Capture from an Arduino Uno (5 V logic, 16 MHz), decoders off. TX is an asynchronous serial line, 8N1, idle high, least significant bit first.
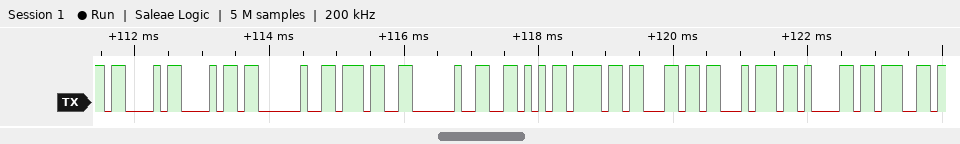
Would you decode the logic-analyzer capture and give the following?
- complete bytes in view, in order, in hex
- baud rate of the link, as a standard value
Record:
0x43 0x68 0x20 0x37 0x20 0x56 0x6F 0x6C 0x74 0x61 0x67
9600 baud
